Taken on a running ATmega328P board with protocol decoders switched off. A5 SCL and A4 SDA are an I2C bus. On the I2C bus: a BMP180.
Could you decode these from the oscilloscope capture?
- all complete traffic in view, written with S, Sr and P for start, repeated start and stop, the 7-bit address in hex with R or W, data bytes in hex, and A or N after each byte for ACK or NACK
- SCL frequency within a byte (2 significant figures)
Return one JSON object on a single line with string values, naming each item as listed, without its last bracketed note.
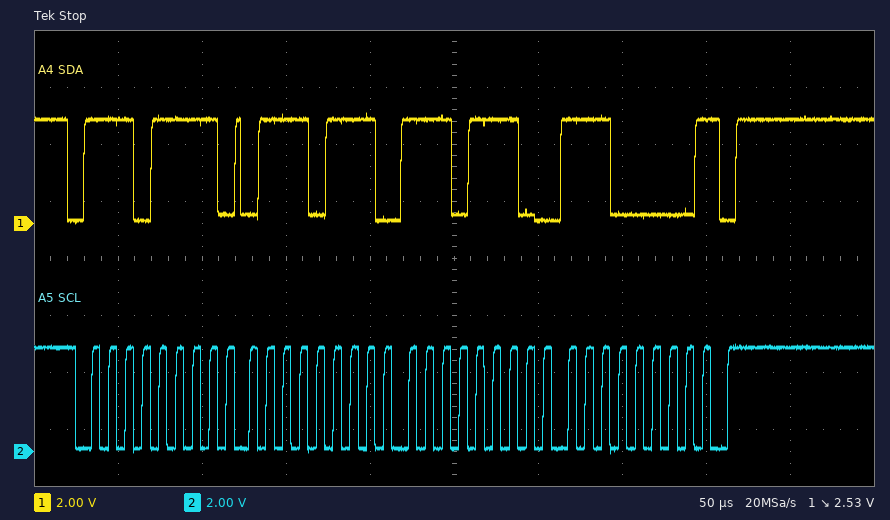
{"all complete traffic in view, written with S, Sr and P for start, repeated start and stop, the 7-bit address in hex with R or W, data bytes in hex, and A or N after each byte for ACK or NACK": "S 77R A 77 A EE A E0 N P", "SCL frequency within a byte": "100 kHz"}
